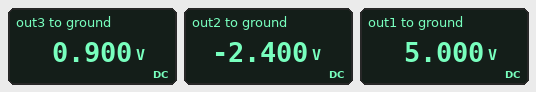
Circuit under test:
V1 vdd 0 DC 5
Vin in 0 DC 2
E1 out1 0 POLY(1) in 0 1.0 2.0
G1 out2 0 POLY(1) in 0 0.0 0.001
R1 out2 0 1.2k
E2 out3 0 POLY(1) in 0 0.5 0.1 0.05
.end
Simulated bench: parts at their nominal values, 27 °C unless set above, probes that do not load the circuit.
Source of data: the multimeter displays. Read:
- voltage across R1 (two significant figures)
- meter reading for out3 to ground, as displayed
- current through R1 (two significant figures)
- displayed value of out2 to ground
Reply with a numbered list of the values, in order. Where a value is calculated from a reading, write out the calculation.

1. 0 V - (-2.4 V) = 2.4 V
2. 0.900 V
3. (0 V - (-2.4 V)) / 1.2 kΩ = 2.0 mA
4. -2.400 V
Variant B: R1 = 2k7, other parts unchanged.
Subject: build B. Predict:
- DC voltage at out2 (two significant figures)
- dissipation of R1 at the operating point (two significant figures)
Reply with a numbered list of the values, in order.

1. -5.4 V
2. 11 mW
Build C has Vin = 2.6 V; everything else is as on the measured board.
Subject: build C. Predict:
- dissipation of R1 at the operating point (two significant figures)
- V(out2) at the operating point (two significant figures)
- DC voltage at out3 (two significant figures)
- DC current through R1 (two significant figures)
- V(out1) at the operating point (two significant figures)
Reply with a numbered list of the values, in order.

1. 8.1 mW
2. -3.1 V
3. 1.1 V
4. 2.6 mA
5. 6.2 V
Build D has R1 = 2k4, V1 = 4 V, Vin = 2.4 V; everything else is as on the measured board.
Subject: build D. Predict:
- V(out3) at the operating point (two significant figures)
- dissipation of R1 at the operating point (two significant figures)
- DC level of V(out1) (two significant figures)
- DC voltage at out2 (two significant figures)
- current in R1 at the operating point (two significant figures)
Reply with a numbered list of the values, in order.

1. 1.0 V
2. 14 mW
3. 5.8 V
4. -5.8 V
5. 2.4 mA
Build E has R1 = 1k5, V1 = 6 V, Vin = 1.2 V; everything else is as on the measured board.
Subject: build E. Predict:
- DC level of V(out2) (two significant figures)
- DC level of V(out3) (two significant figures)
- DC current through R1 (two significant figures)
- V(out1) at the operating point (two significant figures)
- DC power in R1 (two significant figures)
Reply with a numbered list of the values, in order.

1. -1.8 V
2. 690 mV
3. 1.2 mA
4. 3.4 V
5. 2.2 mW
